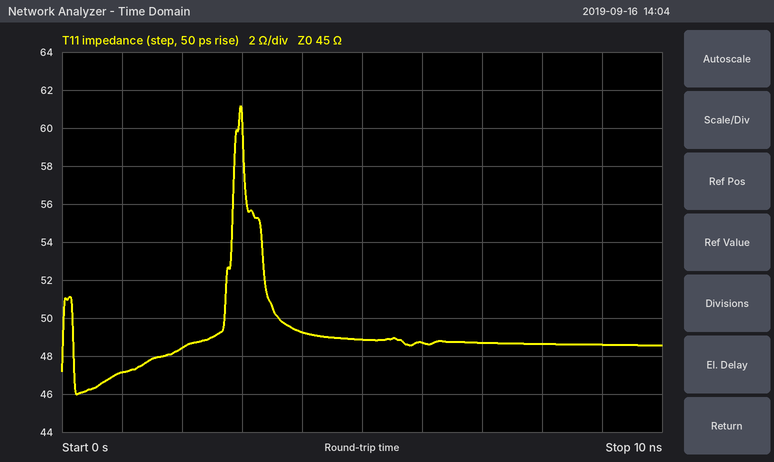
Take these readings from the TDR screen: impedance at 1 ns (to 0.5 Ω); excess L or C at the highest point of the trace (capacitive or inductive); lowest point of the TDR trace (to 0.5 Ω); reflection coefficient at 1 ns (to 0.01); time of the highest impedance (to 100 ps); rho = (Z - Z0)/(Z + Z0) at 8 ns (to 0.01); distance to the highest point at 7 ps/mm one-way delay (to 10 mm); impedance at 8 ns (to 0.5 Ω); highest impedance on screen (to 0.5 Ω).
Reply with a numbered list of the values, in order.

1. 47.0 Ω
2. inductive
3. 46.0 Ω
4. +0.02
5. 3.0 ns
6. +0.04
7. 210 mm
8. 48.5 Ω
9. 61.0 Ω
